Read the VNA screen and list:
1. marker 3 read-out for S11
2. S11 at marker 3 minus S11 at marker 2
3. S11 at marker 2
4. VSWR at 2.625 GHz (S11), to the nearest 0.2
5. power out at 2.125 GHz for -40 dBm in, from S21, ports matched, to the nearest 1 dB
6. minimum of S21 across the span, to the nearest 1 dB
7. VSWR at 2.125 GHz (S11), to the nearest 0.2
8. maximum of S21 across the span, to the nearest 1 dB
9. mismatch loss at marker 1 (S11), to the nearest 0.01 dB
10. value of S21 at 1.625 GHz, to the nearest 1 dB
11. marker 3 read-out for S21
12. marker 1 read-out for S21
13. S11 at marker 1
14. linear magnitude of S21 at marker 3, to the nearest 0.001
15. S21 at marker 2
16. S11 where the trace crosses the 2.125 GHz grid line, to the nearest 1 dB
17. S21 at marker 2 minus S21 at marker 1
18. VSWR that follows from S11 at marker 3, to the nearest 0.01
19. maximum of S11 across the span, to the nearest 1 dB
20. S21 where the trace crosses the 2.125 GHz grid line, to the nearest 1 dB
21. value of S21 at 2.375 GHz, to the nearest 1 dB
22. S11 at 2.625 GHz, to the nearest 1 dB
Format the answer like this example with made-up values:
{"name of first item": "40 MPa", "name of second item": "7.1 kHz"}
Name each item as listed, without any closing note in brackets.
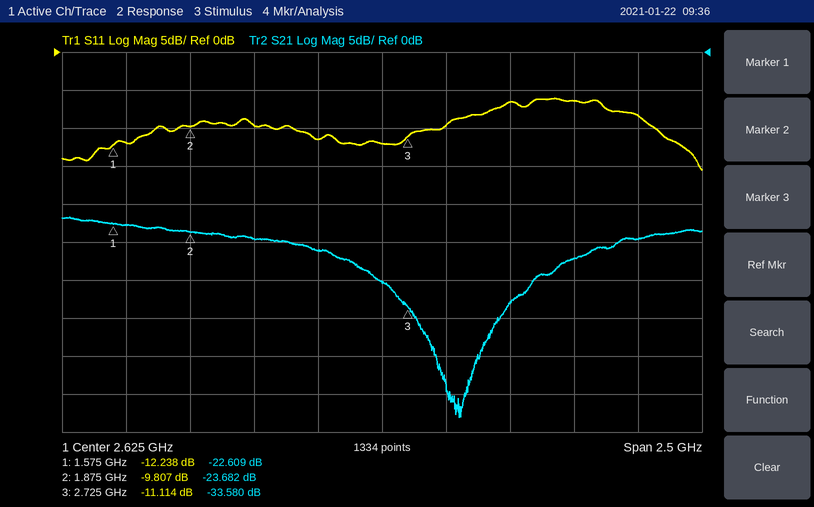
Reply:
{"marker 3 read-out for S11": "-11.114 dB", "S11 at marker 3 minus S11 at marker 2": "-1.307 dB", "S11 at marker 2": "-9.807 dB", "VSWR at 2.625 GHz (S11), to the nearest 0.2": "1.6", "power out at 2.125 GHz for -40 dBm in, from S21, ports matched, to the nearest 1 dB": "-65 dBm", "minimum of S21 across the span, to the nearest 1 dB": "-48 dB", "VSWR at 2.125 GHz (S11), to the nearest 0.2": "2.0", "maximum of S21 across the span, to the nearest 1 dB": "-22 dB", "mismatch loss at marker 1 (S11), to the nearest 0.01 dB": "0.27 dB", "value of S21 at 1.625 GHz, to the nearest 1 dB": "-23 dB", "marker 3 read-out for S21": "-33.580 dB", "marker 1 read-out for S21": "-22.609 dB", "S11 at marker 1": "-12.238 dB", "linear magnitude of S21 at marker 3, to the nearest 0.001": "0.021", "S21 at marker 2": "-23.682 dB", "S11 where the trace crosses the 2.125 GHz grid line, to the nearest 1 dB": "-10 dB", "S21 at marker 2 minus S21 at marker 1": "-1.073 dB", "VSWR that follows from S11 at marker 3, to the nearest 0.01": "1.77", "maximum of S11 across the span, to the nearest 1 dB": "-6 dB", "S21 where the trace crosses the 2.125 GHz grid line, to the nearest 1 dB": "-25 dB", "value of S21 at 2.375 GHz, to the nearest 1 dB": "-26 dB", "S11 at 2.625 GHz, to the nearest 1 dB": "-12 dB"}
